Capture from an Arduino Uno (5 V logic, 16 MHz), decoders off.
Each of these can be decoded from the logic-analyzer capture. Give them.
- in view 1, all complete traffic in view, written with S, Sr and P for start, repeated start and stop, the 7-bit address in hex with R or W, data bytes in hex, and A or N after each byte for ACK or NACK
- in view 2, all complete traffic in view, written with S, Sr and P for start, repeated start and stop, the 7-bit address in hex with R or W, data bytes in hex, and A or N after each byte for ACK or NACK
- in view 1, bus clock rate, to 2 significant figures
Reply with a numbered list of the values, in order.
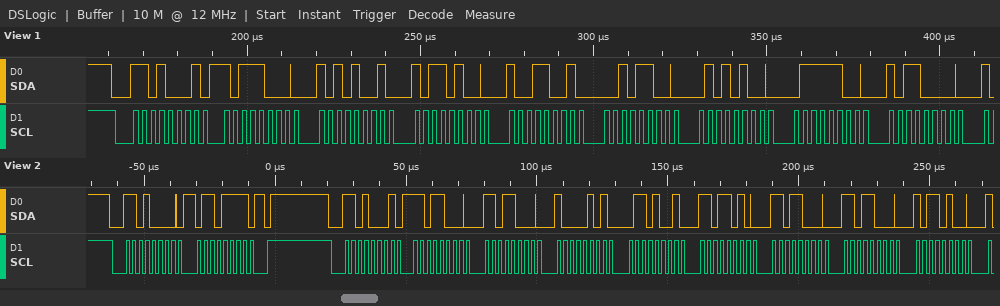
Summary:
1. S 68R A B8 A A9 A B4 A 99 A 2C A 54 A 7C A B0 A
2. S 68W A 6F A P S 68R A D8 A D8 A 85 A 69 A DA A D8 A D8 A B4 A
3. 400 kHz
